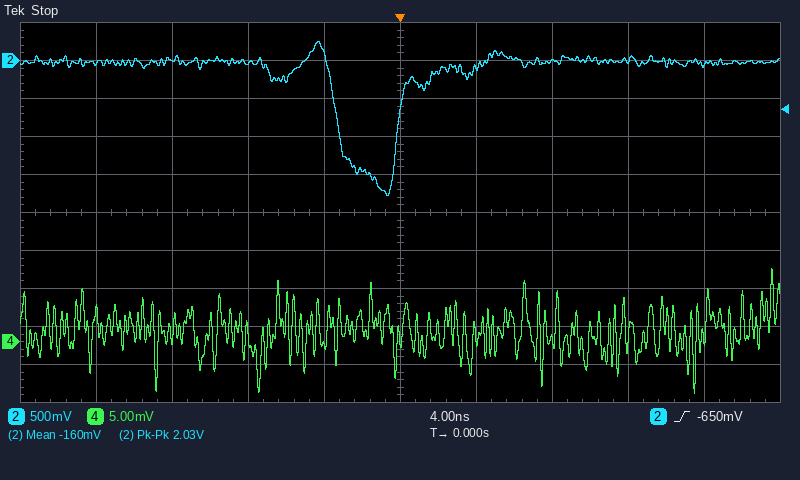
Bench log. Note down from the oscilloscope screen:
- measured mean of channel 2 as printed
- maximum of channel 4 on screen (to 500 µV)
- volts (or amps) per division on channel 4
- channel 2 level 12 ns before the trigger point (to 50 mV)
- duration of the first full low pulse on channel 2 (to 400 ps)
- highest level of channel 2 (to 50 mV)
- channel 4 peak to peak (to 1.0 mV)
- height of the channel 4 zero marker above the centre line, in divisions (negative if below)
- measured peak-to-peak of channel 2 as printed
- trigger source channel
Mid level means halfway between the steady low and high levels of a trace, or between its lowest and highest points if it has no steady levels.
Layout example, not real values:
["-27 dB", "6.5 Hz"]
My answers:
["-160 mV", "9.5 mV", "5 mV", "0 mV", "3.2 ns", "250 mV", "16.0 mV", "-3.4 div", "2.03 V", "channel 2"]
